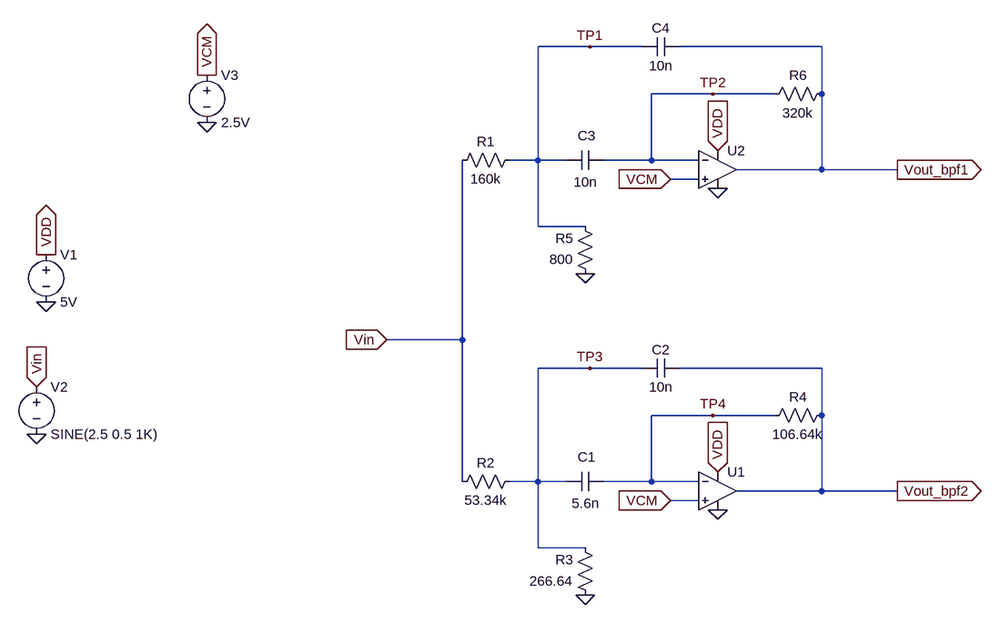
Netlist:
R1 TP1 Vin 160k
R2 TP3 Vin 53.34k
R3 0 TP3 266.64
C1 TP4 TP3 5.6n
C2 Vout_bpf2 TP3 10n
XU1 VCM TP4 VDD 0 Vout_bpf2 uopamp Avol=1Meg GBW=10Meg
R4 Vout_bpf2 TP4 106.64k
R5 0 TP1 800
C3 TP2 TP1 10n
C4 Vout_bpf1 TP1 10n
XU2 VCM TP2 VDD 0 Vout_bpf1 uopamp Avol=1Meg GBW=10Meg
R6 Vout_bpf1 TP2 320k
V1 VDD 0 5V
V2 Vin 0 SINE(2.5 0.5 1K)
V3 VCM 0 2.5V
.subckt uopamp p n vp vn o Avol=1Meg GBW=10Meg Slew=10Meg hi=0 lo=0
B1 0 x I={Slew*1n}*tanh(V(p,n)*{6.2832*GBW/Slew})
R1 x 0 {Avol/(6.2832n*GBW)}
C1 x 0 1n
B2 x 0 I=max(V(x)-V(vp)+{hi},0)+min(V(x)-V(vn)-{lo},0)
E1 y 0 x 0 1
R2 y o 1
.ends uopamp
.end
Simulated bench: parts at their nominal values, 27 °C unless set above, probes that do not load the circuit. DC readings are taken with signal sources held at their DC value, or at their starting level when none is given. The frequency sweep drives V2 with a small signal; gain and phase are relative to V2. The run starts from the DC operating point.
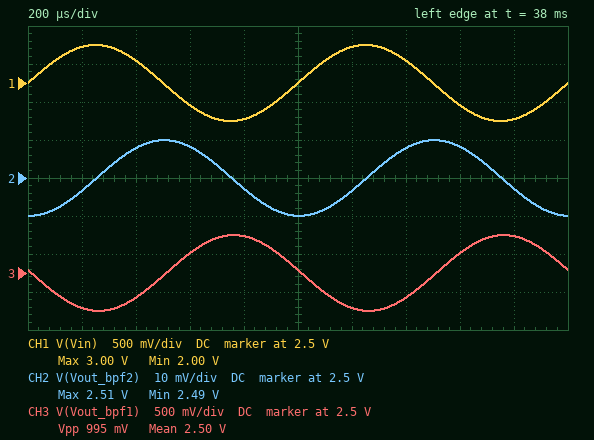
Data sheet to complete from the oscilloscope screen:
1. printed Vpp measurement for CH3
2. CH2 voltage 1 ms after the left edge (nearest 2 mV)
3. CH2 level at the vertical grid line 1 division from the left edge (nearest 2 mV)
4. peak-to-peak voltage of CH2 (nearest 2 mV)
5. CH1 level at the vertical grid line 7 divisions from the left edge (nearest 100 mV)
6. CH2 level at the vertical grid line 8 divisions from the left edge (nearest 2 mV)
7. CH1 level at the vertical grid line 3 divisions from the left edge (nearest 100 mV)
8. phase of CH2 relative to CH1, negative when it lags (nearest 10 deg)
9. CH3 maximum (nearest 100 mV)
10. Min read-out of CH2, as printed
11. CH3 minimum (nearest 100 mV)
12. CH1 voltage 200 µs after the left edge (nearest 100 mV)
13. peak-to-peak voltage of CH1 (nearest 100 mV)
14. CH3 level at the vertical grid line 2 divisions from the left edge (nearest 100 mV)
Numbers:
995 mV
2.490 V
2.496 V
20 mV
2.8 V
2.508 V
2.2 V
-90 deg
3.0 V
2.49 V
2.0 V
3.0 V
1.0 V
2.2 V
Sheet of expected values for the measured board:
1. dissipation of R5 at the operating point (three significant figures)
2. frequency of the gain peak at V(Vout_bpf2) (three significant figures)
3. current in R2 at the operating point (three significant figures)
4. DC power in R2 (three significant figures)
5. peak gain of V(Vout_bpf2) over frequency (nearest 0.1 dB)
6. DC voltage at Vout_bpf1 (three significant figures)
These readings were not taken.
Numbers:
193 nW
3.99 kHz
46.6 µA
116 µW
-2.9 dB
2.50 V
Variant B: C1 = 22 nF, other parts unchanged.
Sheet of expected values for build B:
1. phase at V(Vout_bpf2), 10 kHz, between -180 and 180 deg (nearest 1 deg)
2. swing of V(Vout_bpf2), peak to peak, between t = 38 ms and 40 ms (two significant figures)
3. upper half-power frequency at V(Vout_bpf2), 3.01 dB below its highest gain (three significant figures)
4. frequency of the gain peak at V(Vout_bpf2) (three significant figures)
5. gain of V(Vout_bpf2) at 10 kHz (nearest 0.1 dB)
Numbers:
91 deg
97 mV
2.12 kHz
2.01 kHz
-30.2 dB
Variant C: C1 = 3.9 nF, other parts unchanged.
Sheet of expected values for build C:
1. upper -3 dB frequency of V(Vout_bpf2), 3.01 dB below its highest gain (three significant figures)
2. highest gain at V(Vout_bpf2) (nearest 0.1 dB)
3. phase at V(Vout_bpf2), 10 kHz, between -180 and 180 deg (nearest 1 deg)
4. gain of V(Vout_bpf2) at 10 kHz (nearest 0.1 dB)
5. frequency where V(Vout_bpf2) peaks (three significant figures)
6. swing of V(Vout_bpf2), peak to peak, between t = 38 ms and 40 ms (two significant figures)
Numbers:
5.05 kHz
-5.0 dB
94 deg
-28.3 dB
4.78 kHz
14 mV
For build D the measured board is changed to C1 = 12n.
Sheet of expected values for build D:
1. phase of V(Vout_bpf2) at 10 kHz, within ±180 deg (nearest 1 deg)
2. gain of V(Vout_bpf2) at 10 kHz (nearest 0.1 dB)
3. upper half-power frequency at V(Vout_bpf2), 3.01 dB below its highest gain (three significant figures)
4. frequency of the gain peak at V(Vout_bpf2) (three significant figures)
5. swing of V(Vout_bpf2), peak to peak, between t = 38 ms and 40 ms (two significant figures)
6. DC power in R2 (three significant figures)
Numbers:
92 deg
-29.9 dB
2.86 kHz
2.72 kHz
46 mV
116 µW
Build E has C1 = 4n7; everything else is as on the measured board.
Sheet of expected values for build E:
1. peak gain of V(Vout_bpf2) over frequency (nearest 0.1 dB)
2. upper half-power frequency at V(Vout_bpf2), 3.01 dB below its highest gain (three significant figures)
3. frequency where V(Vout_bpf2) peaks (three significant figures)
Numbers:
-3.9 dB
4.59 kHz
4.35 kHz
